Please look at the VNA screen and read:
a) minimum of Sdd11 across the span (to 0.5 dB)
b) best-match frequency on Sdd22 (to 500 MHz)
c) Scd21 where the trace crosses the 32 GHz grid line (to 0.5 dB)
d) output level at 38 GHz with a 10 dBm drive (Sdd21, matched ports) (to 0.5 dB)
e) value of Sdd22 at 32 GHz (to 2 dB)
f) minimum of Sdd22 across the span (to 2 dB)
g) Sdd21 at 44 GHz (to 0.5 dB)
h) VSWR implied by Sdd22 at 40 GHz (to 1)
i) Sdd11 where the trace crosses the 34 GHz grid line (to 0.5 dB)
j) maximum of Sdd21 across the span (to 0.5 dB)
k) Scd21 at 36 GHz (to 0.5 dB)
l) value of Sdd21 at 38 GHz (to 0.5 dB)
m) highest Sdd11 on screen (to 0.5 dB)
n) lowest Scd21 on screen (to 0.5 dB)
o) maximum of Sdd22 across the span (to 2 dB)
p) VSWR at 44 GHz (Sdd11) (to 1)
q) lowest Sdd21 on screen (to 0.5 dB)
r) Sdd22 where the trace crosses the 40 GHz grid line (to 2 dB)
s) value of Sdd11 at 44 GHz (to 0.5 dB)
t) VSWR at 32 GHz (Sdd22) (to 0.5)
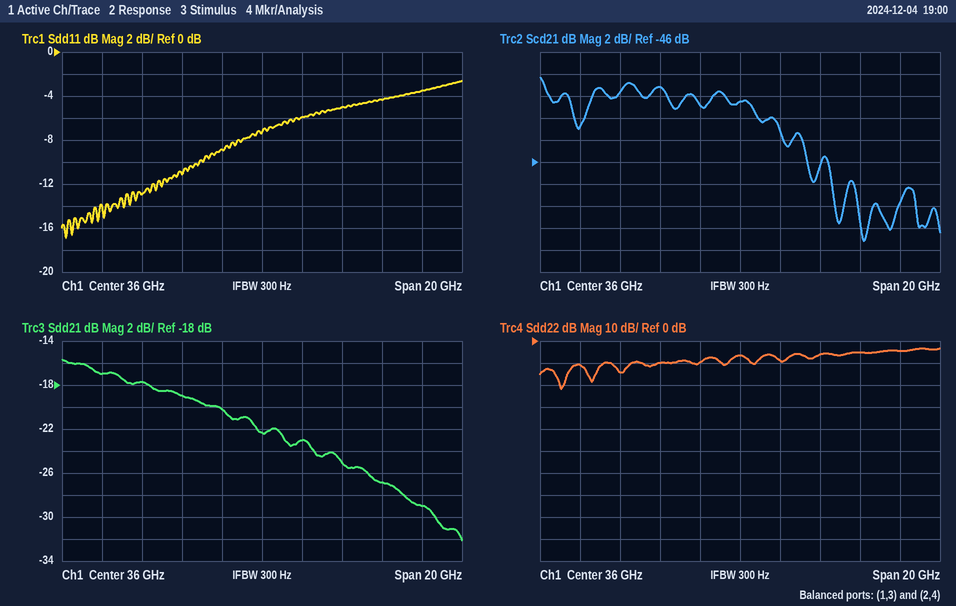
-17.0 dB
27.0 GHz
-39.0 dB
-13.0 dBm
-10 dB
-22 dB
-29.0 dB
3
-9.0 dB
-15.5 dB
-40.5 dB
-23.0 dB
-2.5 dB
-53.0 dB
-4 dB
5
-32.0 dB
-6 dB
-3.5 dB
2.0
